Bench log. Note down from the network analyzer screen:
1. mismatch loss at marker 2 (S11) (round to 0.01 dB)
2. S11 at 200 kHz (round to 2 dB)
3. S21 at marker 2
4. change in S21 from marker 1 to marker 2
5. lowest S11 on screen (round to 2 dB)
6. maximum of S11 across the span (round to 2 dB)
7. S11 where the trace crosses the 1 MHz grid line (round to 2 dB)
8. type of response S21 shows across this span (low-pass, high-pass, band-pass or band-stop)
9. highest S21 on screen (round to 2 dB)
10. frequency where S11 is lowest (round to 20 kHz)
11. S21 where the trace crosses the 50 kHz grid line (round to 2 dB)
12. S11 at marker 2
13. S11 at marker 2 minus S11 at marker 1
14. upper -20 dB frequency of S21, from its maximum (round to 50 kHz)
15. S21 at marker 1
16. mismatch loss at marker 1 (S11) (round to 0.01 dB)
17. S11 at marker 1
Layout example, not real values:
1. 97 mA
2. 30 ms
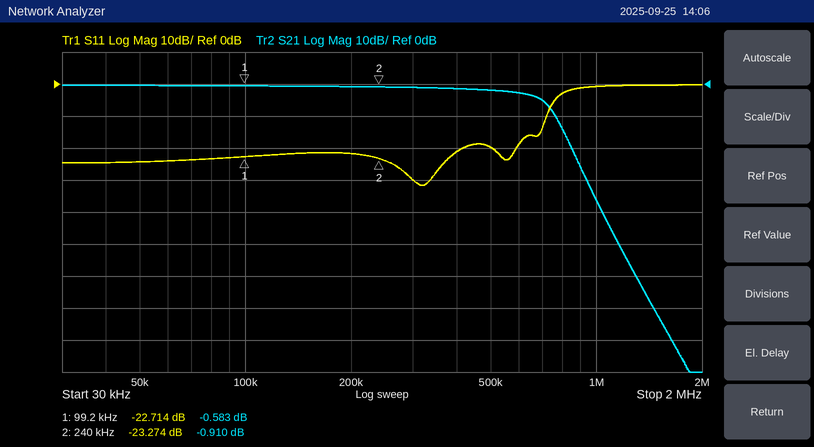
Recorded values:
1. 0.02 dB
2. -22 dB
3. -0.910 dB
4. -0.327 dB
5. -32 dB
6. 0 dB
7. 0 dB
8. low-pass
9. 0 dB
10. 320 kHz
11. 0 dB
12. -23.274 dB
13. -0.560 dB
14. 850 kHz
15. -0.583 dB
16. 0.02 dB
17. -22.714 dB
